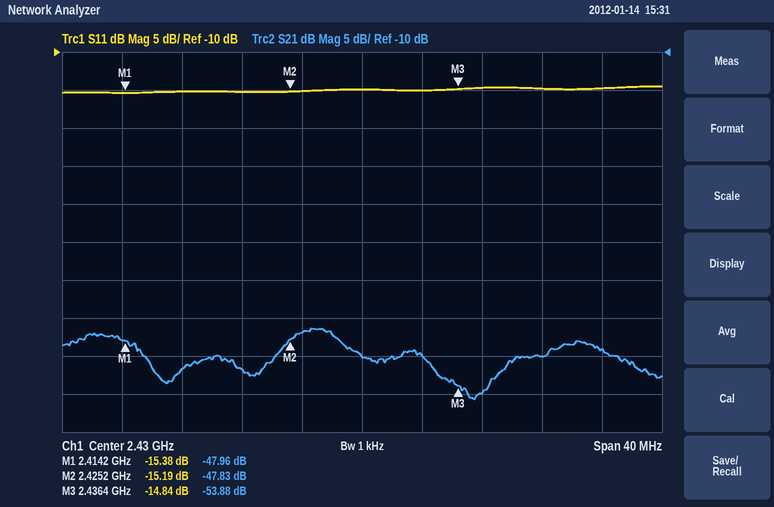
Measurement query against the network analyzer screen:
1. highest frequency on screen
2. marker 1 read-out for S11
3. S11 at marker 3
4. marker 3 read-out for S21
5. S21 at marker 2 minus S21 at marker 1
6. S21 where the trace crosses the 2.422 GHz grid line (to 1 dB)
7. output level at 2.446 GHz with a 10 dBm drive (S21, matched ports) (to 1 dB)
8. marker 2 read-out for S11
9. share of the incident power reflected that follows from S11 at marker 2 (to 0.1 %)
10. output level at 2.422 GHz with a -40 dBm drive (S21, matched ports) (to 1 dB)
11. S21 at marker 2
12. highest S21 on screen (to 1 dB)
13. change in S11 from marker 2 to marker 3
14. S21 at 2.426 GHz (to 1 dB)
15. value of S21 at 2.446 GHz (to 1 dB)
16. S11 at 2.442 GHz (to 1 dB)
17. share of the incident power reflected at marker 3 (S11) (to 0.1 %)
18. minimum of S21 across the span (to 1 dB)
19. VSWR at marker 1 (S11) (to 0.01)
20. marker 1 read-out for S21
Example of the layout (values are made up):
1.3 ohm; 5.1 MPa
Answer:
2.45 GHz; -15.38 dB; -14.84 dB; -53.88 dB; 0.13 dB; -52 dB; -39 dBm; -15.19 dB; 3.0 %; -92 dBm; -47.83 dB; -46 dB; 0.35 dB; -47 dB; -49 dB; -15 dB; 3.3 %; -56 dB; 1.41; -47.96 dB
